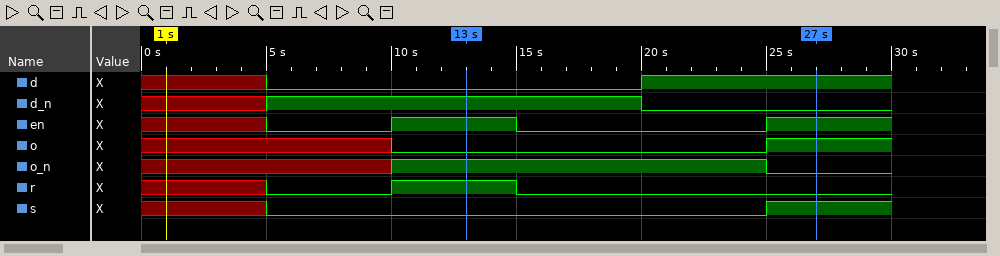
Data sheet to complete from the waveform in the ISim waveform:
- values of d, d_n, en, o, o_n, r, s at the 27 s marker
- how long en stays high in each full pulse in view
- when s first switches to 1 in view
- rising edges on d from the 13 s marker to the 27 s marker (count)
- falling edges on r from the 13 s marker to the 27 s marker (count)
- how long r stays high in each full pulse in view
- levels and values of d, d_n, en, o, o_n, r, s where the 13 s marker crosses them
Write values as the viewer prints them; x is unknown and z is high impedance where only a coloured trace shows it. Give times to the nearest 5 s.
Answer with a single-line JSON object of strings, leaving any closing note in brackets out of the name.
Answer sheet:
{"values of d, d_n, en, o, o_n, r, s at the 27 s marker": "d=1, d_n=0, en=1, o=1, o_n=0, r=0, s=1", "how long en stays high in each full pulse in view": "5 s", "when s first switches to 1 in view": "25 s", "rising edges on d from the 13 s marker to the 27 s marker": "1", "falling edges on r from the 13 s marker to the 27 s marker": "1", "how long r stays high in each full pulse in view": "5 s", "levels and values of d, d_n, en, o, o_n, r, s where the 13 s marker crosses them": "d=0, d_n=1, en=1, o=0, o_n=1, r=1, s=0"}
